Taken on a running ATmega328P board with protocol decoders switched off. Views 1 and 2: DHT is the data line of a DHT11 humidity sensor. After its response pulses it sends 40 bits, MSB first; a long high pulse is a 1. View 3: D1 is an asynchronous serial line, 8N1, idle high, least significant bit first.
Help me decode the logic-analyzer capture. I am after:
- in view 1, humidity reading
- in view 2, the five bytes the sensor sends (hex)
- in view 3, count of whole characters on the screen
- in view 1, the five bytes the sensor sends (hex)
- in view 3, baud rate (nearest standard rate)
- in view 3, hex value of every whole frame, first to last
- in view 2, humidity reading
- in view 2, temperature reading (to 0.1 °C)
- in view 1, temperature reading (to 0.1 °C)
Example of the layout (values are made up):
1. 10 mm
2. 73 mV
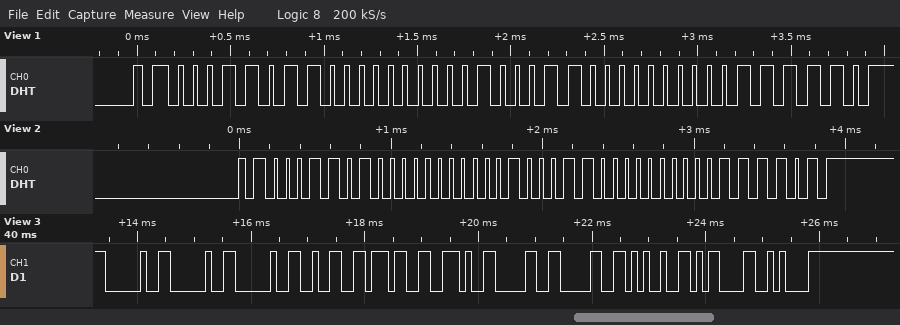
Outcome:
1. 27 %
2. 1A 00 23 00 3D
3. 11
4. 1B 00 23 00 3E
5. 9600 baud
6. 20 20 20 32 37 2E 30 30 25 0D 0A
7. 26 %
8. 35.0 °C
9. 35.0 °C
